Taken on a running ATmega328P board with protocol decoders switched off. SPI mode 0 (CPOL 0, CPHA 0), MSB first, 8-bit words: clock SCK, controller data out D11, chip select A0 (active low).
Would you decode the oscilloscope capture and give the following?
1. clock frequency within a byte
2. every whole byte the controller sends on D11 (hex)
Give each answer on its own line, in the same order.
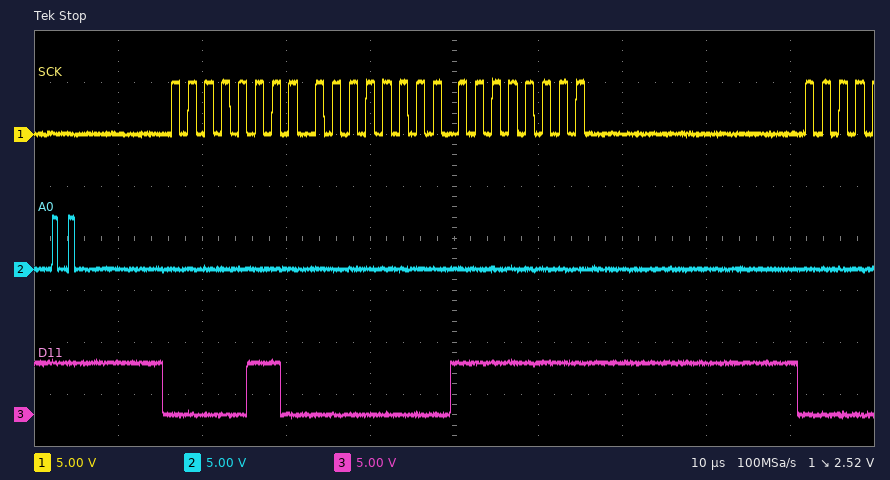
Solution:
500 kHz
06 00 FF
